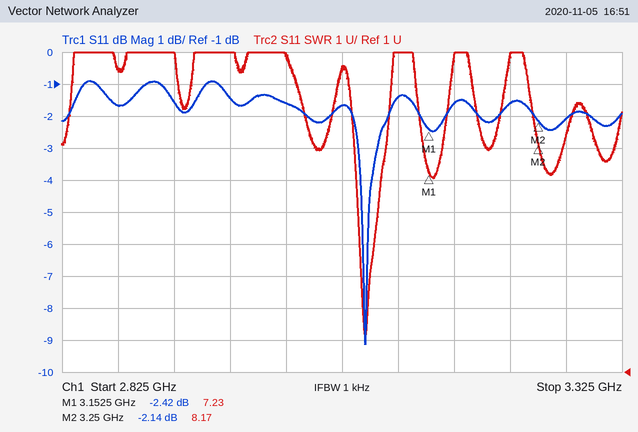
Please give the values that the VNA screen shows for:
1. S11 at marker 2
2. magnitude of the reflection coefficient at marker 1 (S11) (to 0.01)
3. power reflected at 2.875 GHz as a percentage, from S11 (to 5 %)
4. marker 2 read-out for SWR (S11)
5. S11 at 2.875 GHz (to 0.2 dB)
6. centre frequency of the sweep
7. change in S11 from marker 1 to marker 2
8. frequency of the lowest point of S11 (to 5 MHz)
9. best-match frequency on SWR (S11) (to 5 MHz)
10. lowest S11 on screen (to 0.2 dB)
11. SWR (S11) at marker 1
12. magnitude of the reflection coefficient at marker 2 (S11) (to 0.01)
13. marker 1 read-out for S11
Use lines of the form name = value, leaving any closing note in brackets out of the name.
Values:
S11 at marker 2 = -2.14 dB
magnitude of the reflection coefficient at marker 1 (S11) = 0.76
power reflected at 2.875 GHz as a percentage, from S11 = 70 %
marker 2 read-out for SWR = 8.17
S11 at 2.875 GHz = -1.6 dB
centre frequency of the sweep = 3.075 GHz
change in S11 from marker 1 to marker 2 = 0.28 dB
frequency of the lowest point of S11 = 3.095 GHz
best-match frequency on SWR (S11) = 3.095 GHz
lowest S11 on screen = -9.2 dB
SWR (S11) at marker 1 = 7.23
magnitude of the reflection coefficient at marker 2 (S11) = 0.78
marker 1 read-out for S11 = -2.42 dB
